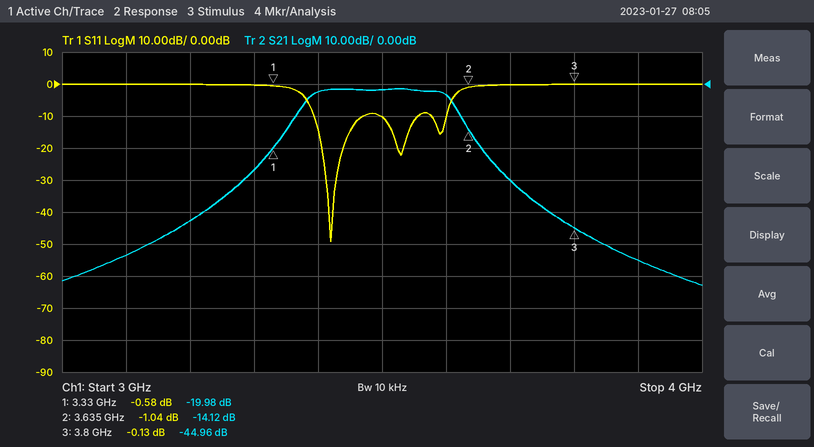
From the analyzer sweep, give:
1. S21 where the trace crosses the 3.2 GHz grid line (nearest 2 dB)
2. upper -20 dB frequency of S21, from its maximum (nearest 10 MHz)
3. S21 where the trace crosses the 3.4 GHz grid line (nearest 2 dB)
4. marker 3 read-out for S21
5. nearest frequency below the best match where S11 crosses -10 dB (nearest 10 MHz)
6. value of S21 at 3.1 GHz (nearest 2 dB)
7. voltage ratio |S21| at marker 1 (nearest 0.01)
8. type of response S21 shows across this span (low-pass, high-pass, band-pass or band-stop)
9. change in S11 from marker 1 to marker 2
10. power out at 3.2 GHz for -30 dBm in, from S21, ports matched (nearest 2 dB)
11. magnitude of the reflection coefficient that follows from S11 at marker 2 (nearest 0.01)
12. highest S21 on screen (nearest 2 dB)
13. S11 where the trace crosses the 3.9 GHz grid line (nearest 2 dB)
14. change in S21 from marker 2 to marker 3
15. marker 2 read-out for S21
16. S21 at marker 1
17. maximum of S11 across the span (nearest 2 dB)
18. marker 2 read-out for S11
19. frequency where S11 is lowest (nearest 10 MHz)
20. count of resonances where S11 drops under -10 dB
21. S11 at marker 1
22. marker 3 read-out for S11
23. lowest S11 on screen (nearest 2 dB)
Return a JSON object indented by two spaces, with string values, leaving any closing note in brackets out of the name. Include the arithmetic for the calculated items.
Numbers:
{
  "S21 where the trace crosses the 3.2 GHz grid line": "-42 dB",
  "upper -20 dB frequency of S21, from its maximum": "3.66 GHz",
  "S21 where the trace crosses the 3.4 GHz grid line": "-2 dB",
  "marker 3 read-out for S21": "-44.96 dB",
  "nearest frequency below the best match where S11 crosses -10 dB": "3.39 GHz",
  "value of S21 at 3.1 GHz": "-54 dB",
  "voltage ratio |S21| at marker 1": "10^(-19.98/20) ≈ 0.10",
  "type of response S21 shows across this span": "band-pass",
  "change in S11 from marker 1 to marker 2": "-1.04 − (-0.58) = -0.46 dB",
  "power out at 3.2 GHz for -30 dBm in, from S21, ports matched": "-30 dBm + (-42 dB) = -72 dBm",
  "magnitude of the reflection coefficient that follows from S11 at marker 2": "10^(-1.04/20) ≈ 0.89",
  "highest S21 on screen": "-2 dB",
  "S11 where the trace crosses the 3.9 GHz grid line": "0 dB",
  "change in S21 from marker 2 to marker 3": "-44.96 − (-14.12) = -30.84 dB",
  "marker 2 read-out for S21": "-14.12 dB",
  "S21 at marker 1": "-19.98 dB",
  "maximum of S11 across the span": "0 dB",
  "marker 2 read-out for S11": "-1.04 dB",
  "frequency where S11 is lowest": "3.42 GHz",
  "count of resonances where S11 drops under -10 dB": "3",
  "S11 at marker 1": "-0.58 dB",
  "marker 3 read-out for S11": "-0.13 dB",
  "lowest S11 on screen": "-50 dB"
}
